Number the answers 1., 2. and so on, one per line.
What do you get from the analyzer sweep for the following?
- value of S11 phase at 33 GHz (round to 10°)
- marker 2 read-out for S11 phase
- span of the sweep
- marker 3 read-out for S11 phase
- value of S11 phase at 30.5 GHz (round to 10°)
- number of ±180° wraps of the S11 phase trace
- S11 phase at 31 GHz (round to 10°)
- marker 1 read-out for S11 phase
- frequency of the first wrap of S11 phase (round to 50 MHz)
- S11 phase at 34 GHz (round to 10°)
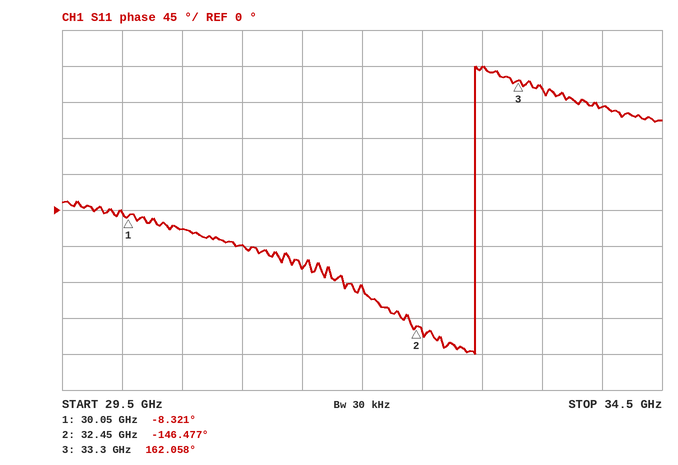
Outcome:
1. 180°
2. -146.477°
3. 5 GHz
4. 162.058°
5. -20°
6. 1
7. -40°
8. -8.321°
9. 32.95 GHz
10. 130°
